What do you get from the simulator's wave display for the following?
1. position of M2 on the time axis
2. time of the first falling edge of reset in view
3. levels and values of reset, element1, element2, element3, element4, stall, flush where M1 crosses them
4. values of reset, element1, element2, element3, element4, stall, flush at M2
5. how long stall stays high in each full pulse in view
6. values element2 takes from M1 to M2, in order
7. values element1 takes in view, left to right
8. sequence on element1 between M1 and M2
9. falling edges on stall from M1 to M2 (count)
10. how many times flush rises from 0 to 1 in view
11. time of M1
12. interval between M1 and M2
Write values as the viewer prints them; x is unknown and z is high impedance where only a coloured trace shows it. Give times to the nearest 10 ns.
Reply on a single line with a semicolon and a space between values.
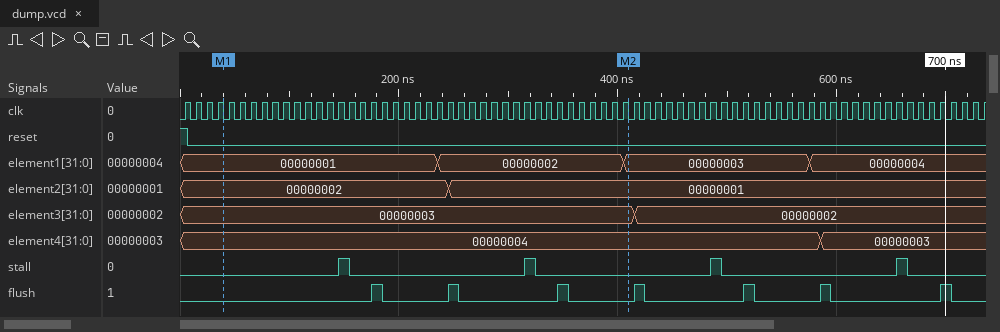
410 ns; 10 ns; reset=0, element1=00000001, element2=00000002, element3=00000003, element4=00000004, stall=0, flush=0; reset=0, element1=00000003, element2=00000001, element3=00000003, element4=00000004, stall=0, flush=0; 10 ns, 10 ns, 10 ns, 10 ns; 00000002, 00000001; 00000001, 00000002, 00000003, 00000004; 00000001, 00000002, 00000003; 2; 7; 40 ns; 370 ns
